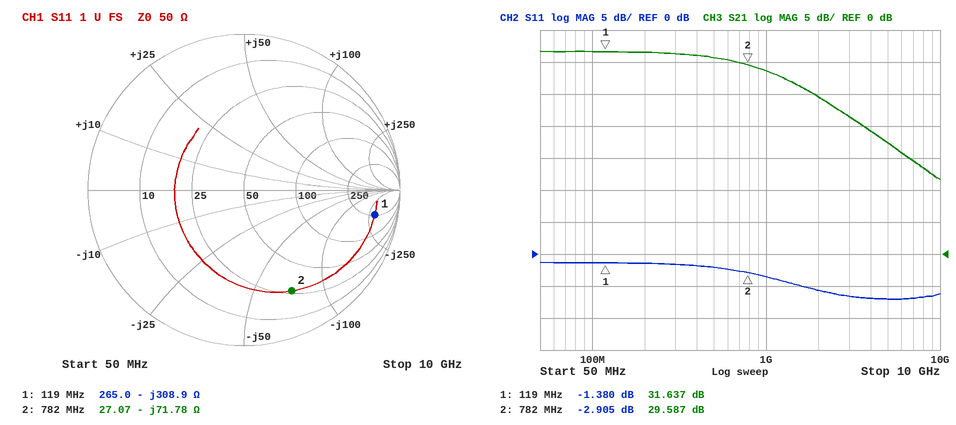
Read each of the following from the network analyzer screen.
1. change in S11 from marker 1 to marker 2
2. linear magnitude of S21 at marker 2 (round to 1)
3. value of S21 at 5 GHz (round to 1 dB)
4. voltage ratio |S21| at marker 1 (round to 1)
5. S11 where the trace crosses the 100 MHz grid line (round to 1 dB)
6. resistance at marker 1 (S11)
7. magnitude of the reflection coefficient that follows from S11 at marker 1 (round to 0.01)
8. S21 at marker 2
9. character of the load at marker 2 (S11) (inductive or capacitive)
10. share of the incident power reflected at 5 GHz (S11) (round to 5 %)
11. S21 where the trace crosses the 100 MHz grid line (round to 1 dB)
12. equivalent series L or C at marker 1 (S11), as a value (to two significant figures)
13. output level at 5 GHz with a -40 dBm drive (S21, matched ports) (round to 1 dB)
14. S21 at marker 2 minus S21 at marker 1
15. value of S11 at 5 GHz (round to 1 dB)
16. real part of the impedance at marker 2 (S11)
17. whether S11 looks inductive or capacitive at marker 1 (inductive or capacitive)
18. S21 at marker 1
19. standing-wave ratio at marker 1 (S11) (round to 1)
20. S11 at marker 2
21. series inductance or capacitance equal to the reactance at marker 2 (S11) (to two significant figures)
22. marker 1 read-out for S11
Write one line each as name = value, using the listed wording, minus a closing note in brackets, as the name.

change in S11 from marker 1 to marker 2 = -1.525 dB
linear magnitude of S21 at marker 2 = 30
value of S21 at 5 GHz = 17 dB
voltage ratio |S21| at marker 1 = 38
S11 where the trace crosses the 100 MHz grid line = -1 dB
resistance at marker 1 = 265.0 Ω
magnitude of the reflection coefficient that follows from S11 at marker 1 = 0.85
S21 at marker 2 = 29.587 dB
character of the load at marker 2 (S11) = capacitive
share of the incident power reflected at 5 GHz (S11) = 20 %
S21 where the trace crosses the 100 MHz grid line = 32 dB
equivalent series L or C at marker 1 (S11), as a value = 4.3 pF
output level at 5 GHz with a -40 dBm drive (S21, matched ports) = -23 dBm
S21 at marker 2 minus S21 at marker 1 = -2.050 dB
value of S11 at 5 GHz = -7 dB
real part of the impedance at marker 2 = 27.07 Ω
whether S11 looks inductive or capacitive at marker 1 = capacitive
S21 at marker 1 = 31.637 dB
standing-wave ratio at marker 1 (S11) = 13
S11 at marker 2 = -2.905 dB
series inductance or capacitance equal to the reactance at marker 2 (S11) = 2.8 pF
marker 1 read-out for S11 = -1.380 dB
